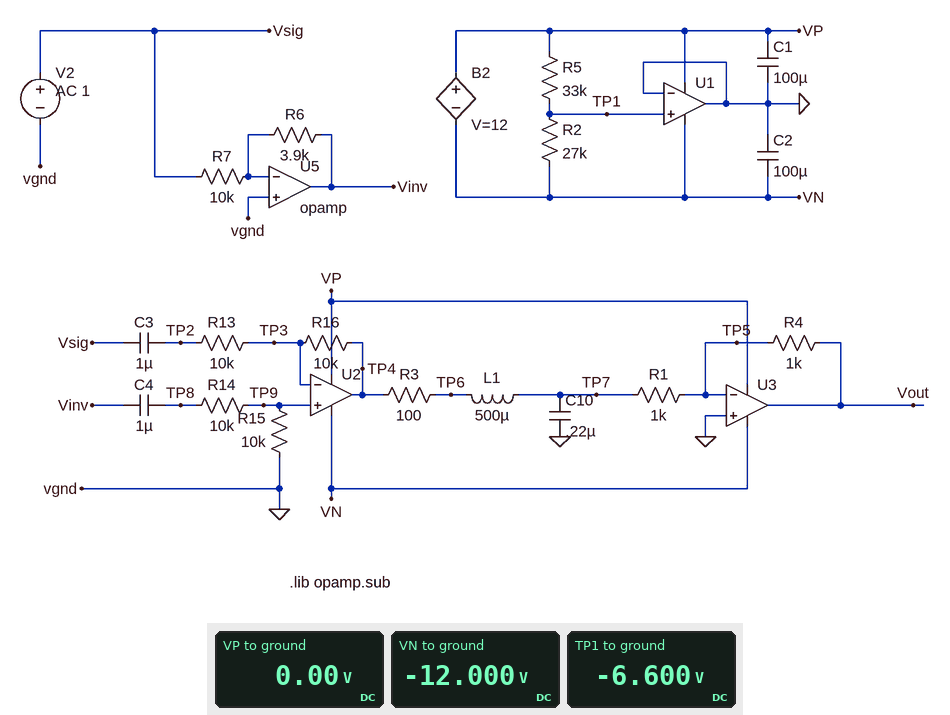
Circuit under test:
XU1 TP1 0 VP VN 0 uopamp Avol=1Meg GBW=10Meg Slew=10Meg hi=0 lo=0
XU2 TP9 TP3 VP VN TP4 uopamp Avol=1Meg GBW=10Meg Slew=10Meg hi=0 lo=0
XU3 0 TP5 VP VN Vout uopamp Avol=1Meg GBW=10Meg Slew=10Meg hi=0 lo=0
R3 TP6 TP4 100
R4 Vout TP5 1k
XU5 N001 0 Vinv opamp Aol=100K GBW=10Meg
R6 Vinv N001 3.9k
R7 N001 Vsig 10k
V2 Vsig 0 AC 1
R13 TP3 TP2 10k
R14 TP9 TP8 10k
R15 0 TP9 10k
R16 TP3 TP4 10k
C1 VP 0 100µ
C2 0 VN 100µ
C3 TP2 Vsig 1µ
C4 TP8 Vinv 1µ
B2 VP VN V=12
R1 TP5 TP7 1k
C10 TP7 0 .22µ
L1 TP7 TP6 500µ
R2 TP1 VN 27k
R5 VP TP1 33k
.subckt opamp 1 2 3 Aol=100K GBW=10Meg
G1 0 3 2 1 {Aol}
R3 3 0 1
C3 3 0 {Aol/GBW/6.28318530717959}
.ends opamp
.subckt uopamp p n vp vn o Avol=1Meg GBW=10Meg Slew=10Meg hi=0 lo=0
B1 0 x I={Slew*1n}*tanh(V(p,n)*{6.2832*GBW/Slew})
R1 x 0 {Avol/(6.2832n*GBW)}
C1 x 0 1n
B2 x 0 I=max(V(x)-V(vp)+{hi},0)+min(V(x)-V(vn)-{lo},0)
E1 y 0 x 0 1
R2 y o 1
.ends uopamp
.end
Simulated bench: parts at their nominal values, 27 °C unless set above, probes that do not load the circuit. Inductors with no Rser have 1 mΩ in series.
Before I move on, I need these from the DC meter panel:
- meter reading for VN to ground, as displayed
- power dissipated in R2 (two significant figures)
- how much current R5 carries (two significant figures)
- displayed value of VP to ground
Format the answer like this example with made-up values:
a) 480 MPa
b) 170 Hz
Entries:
a) -12.000 V
b) 1.1 mW
c) 200 µA
d) 0.00 V
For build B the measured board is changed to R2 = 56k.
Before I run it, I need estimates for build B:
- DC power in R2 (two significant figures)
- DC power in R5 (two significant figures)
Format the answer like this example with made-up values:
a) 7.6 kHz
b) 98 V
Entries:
a) 1.0 mW
b) 600 µW
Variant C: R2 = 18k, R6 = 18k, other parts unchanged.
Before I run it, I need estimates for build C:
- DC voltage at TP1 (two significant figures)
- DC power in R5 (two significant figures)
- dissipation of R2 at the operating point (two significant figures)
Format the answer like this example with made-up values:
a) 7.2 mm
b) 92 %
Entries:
a) 4.2 V
b) 1.8 mW
c) 1.0 mW
